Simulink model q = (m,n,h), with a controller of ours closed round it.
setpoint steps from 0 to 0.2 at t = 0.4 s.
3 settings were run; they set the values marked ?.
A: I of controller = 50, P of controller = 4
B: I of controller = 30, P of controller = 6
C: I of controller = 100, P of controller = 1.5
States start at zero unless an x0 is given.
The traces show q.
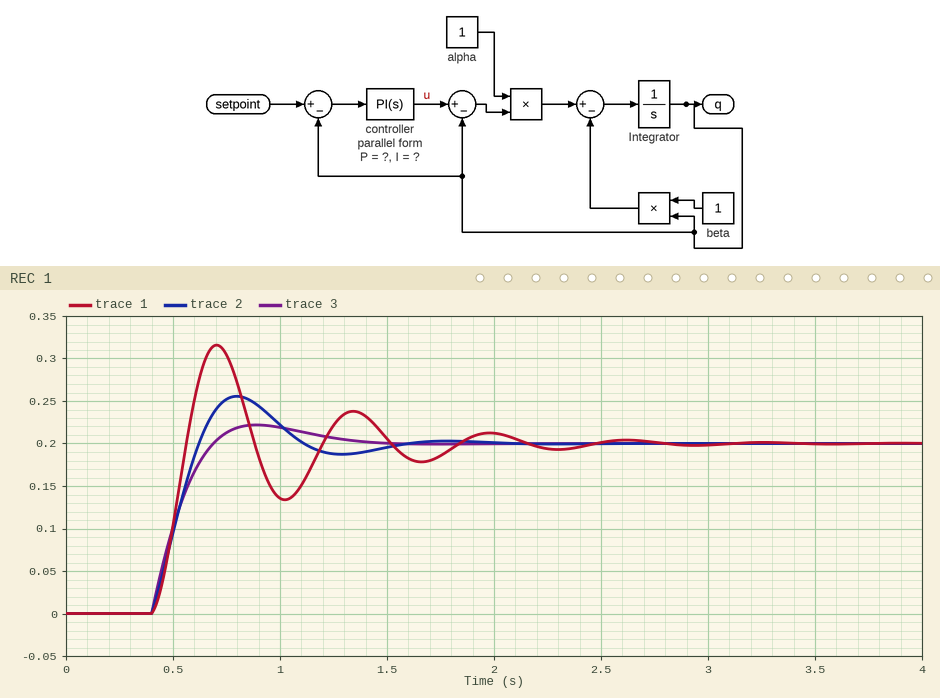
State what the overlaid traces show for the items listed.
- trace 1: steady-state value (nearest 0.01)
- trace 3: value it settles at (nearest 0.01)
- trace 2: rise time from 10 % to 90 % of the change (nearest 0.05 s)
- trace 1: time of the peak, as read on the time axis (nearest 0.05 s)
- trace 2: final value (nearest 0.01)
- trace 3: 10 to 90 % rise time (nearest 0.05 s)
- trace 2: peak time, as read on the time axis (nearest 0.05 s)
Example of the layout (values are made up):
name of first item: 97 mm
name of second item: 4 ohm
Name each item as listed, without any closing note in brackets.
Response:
trace 1: steady-state value: 0.20
trace 3: value it settles at: 0.20
trace 2: rise time from 10 % to 90 % of the change: 0.15 s
trace 1: time of the peak, as read on the time axis: 0.70 s
trace 2: final value: 0.20
trace 3: 10 to 90 % rise time: 0.20 s
trace 2: peak time, as read on the time axis: 0.80 s
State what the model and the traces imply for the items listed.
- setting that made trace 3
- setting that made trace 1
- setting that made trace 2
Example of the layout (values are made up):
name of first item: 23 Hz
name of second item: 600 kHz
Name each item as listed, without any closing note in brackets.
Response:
setting that made trace 3: B
setting that made trace 1: C
setting that made trace 2: A
